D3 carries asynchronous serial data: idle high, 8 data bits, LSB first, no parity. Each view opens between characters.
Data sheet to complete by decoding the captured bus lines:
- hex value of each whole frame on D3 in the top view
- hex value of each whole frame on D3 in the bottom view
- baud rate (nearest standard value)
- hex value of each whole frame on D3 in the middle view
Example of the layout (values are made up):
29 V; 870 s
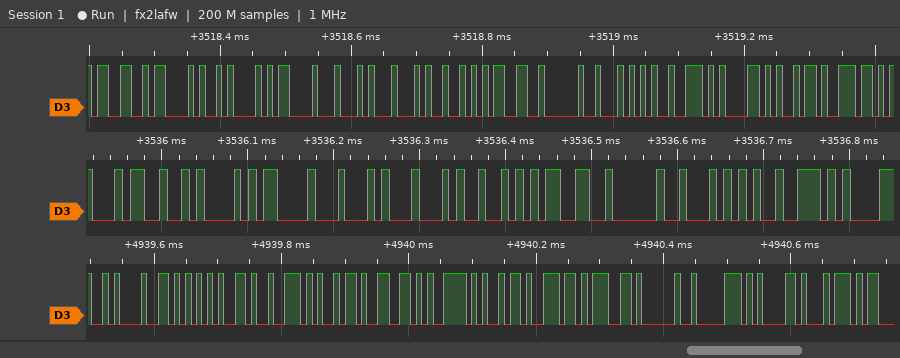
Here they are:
33, 43, 0A, 0D, 44, 44, 52, 33, 20, 54, 72, 61, 69, 6E; 0A, 56, 65, 72, 69, 66, 79, 69, 6E, 67, 20, 70, 61, 74; 115200 baud; 34, 0A, 0D, 44, 44, 52, 33, 20, 54, 72
